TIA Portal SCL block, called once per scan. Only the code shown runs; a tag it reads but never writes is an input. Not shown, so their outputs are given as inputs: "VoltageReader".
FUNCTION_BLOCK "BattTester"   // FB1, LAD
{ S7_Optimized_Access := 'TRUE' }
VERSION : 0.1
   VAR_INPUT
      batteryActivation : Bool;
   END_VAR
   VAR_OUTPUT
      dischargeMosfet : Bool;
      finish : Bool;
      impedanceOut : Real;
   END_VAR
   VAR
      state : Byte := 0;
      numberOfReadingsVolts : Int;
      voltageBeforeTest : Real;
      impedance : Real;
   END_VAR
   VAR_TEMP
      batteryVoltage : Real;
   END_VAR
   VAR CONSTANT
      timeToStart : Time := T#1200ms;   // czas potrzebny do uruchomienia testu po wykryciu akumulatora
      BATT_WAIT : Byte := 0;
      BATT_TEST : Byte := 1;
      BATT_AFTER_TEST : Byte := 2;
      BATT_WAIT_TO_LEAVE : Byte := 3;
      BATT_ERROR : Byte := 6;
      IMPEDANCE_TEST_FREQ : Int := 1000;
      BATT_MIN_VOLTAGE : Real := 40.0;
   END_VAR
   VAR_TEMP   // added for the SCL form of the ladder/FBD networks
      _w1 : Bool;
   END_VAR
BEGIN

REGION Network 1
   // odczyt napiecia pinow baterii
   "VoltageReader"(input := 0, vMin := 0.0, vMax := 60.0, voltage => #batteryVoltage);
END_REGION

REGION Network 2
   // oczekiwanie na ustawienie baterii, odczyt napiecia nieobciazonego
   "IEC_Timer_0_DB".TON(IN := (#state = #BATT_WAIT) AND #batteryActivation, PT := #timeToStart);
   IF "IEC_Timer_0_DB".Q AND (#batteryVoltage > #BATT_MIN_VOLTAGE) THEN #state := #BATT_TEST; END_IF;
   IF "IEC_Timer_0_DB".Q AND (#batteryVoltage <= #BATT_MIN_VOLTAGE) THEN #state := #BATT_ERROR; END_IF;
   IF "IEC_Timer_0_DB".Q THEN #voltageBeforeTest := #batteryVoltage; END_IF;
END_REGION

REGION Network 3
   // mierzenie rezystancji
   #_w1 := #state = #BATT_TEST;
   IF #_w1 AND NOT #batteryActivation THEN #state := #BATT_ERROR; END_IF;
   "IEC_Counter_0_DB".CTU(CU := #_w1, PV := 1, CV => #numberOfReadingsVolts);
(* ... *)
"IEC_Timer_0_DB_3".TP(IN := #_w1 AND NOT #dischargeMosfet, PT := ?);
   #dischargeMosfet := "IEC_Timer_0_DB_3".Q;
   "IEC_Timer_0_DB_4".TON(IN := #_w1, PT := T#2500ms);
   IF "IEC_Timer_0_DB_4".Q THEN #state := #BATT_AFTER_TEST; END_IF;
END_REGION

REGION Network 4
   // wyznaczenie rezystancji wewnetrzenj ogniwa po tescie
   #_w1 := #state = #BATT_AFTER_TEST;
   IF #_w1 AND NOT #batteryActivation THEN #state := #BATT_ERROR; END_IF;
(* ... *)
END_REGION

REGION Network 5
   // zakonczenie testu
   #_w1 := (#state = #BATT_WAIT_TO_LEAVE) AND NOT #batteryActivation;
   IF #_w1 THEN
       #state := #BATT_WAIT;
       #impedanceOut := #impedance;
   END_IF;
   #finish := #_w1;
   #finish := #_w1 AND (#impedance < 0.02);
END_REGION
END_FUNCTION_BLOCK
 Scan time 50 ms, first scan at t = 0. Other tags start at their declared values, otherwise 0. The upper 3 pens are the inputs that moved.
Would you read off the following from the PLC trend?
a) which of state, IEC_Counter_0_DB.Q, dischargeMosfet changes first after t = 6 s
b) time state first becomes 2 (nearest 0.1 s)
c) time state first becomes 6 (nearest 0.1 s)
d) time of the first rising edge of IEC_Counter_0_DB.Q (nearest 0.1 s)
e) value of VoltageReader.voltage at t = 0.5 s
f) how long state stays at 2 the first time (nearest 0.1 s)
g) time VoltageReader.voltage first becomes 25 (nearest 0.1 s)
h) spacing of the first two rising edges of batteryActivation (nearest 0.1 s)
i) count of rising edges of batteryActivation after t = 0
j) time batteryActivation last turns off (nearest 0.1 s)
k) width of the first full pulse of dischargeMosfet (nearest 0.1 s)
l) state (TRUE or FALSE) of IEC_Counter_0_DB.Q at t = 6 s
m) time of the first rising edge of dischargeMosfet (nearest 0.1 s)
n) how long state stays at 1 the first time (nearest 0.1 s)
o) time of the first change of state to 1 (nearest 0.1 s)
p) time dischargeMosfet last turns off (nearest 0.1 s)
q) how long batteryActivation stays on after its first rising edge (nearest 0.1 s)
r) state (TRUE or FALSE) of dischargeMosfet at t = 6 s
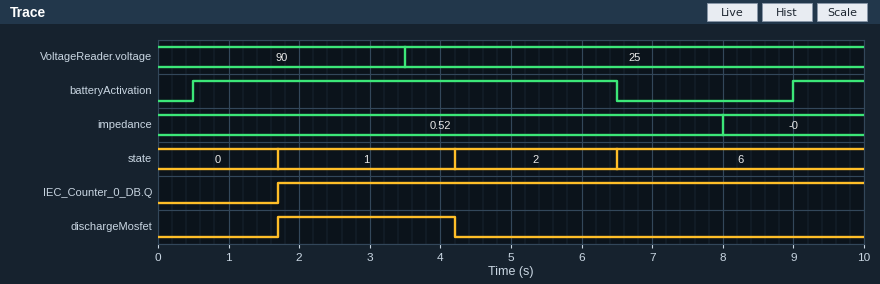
state
4.2 s
6.5 s
1.7 s
90
2.3 s
3.5 s
8.5 s
2
6.5 s
2.5 s
TRUE
1.7 s
2.5 s
1.7 s
4.2 s
6.0 s
FALSE
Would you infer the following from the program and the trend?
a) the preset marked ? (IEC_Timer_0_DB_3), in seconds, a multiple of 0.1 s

2.5 s
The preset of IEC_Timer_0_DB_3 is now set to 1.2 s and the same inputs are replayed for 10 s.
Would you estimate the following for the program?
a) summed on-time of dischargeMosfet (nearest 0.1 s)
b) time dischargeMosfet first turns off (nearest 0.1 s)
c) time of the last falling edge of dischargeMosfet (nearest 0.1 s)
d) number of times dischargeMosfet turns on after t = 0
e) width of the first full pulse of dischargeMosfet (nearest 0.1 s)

3.6 s
2.9 s
5.4 s
3
1.2 s
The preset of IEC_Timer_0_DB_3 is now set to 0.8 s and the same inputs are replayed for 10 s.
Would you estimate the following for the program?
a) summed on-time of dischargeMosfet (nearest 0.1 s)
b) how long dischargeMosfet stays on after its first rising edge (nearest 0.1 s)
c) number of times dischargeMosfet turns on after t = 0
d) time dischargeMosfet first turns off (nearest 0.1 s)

2.4 s
0.8 s
3
2.5 s
